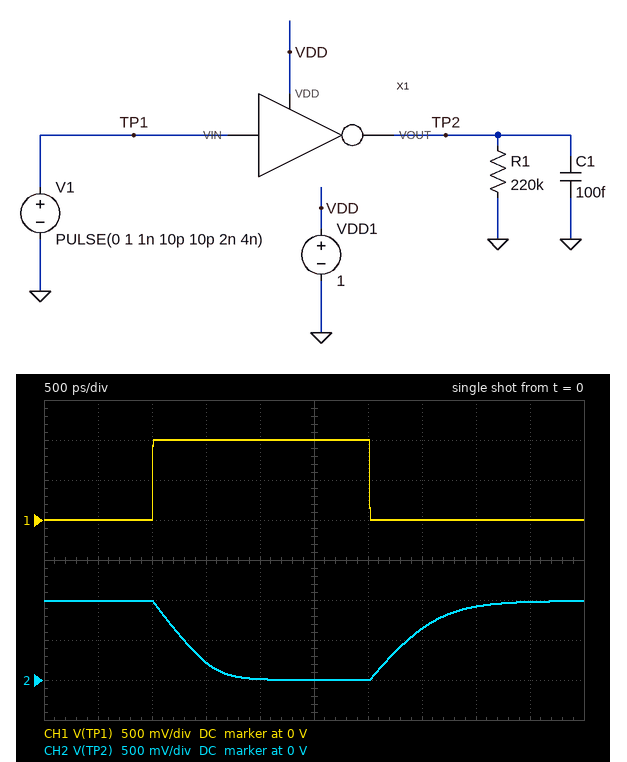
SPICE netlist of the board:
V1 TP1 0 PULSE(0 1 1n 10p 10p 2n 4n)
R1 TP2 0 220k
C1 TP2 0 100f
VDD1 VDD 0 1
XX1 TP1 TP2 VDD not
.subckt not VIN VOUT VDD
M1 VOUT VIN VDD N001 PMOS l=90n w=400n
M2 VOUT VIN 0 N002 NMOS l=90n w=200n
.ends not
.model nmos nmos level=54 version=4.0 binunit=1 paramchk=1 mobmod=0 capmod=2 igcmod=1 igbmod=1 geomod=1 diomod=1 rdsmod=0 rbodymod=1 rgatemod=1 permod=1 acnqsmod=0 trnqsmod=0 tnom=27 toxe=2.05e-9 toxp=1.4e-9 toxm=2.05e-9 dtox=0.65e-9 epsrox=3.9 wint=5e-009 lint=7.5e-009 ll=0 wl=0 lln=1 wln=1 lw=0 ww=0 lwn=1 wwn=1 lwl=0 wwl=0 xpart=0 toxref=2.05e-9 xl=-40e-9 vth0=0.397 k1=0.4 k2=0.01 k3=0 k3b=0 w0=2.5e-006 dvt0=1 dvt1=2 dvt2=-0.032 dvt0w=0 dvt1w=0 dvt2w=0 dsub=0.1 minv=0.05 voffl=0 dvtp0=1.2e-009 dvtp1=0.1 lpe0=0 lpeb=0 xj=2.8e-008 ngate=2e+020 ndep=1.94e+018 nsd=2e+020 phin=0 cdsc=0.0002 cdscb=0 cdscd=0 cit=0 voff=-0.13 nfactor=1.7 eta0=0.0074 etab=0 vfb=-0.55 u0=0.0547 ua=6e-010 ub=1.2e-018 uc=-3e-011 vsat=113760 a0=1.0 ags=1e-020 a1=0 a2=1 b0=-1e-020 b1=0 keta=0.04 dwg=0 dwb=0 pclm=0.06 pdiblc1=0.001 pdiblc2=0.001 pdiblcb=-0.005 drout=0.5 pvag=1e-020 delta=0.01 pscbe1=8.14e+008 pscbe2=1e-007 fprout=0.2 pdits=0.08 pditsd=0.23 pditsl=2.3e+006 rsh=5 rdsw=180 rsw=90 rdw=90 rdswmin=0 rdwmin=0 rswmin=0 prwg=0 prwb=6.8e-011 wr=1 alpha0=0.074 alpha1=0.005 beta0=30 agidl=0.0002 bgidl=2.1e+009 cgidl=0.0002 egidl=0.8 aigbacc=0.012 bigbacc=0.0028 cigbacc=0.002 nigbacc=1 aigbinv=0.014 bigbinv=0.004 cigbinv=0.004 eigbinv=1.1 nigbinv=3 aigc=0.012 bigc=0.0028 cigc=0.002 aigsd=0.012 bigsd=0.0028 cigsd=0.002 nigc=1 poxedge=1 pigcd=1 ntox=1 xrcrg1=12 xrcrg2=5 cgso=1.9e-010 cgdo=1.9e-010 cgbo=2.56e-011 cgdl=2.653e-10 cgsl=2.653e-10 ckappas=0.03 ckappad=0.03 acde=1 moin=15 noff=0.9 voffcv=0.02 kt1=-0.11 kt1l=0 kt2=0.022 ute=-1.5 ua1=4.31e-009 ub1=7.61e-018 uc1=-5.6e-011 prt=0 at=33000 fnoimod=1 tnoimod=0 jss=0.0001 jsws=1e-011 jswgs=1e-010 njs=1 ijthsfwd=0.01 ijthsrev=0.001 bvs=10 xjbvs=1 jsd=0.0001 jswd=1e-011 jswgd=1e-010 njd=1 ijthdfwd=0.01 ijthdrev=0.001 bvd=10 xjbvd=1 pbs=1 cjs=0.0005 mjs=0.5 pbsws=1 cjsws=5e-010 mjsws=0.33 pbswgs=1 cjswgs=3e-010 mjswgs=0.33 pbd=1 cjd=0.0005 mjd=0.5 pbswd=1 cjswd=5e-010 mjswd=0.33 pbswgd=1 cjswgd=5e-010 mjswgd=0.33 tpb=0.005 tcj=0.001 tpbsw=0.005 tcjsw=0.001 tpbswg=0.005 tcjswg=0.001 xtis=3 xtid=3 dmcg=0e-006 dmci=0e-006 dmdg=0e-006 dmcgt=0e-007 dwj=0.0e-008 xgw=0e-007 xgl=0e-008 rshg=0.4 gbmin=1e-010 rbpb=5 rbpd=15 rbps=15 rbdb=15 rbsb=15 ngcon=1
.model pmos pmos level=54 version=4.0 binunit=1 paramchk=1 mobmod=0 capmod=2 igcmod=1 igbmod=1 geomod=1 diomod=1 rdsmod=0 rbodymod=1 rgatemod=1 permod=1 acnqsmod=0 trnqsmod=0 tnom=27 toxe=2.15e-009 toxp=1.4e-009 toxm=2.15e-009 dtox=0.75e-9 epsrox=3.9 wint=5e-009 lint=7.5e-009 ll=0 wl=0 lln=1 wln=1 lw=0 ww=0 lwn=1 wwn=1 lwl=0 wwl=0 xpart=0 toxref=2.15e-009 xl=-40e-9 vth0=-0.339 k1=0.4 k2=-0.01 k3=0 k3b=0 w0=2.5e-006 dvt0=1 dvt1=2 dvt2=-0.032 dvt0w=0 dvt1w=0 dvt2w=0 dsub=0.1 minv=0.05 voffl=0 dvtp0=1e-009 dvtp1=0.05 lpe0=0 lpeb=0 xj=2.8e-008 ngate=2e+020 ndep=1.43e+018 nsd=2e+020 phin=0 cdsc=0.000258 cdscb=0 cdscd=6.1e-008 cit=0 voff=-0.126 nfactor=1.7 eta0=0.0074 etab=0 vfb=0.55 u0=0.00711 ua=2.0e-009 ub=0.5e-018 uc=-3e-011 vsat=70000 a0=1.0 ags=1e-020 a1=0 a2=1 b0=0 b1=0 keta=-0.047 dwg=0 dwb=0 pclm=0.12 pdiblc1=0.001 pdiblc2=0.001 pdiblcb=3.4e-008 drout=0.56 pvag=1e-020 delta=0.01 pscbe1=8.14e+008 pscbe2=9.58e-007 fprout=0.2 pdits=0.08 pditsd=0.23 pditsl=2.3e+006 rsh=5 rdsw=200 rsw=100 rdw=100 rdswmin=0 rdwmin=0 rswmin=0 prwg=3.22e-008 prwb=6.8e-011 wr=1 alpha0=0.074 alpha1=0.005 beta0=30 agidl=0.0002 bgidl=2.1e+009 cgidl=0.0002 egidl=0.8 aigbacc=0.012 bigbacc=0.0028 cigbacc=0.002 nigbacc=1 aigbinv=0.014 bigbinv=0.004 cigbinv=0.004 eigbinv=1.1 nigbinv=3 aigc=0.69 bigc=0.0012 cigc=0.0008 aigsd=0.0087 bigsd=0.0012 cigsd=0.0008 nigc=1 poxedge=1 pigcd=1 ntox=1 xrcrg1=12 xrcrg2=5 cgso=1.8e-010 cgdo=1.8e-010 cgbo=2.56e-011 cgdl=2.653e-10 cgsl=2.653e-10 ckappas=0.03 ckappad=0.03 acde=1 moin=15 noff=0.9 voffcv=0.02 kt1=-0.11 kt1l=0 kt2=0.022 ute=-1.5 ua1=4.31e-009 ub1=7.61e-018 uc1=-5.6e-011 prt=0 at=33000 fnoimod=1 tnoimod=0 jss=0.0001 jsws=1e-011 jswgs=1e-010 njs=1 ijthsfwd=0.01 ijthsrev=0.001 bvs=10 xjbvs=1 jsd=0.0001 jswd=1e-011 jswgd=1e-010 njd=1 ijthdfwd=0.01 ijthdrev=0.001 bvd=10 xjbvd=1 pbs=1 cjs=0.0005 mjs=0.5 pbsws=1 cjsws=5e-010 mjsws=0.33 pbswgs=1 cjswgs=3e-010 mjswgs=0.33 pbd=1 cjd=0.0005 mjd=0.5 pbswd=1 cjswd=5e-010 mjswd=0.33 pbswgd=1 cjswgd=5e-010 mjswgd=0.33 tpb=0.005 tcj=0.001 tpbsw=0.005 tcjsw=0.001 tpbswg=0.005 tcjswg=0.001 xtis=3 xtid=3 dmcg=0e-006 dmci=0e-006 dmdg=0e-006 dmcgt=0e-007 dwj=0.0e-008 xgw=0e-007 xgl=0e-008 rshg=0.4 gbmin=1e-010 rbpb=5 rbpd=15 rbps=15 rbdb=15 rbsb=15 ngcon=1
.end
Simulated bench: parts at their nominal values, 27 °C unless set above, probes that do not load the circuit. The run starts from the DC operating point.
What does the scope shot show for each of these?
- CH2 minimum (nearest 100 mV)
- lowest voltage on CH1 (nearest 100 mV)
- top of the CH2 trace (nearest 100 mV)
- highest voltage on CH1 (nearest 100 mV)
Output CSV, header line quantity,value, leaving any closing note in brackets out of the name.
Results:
quantity,value
CH2 minimum,0 V
lowest voltage on CH1,0 V
top of the CH2 trace,1.0 V
highest voltage on CH1,1.0 V
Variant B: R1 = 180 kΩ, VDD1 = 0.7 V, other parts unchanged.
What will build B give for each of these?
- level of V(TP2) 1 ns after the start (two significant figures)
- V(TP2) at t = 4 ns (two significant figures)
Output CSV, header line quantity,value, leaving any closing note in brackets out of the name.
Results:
quantity,value
level of V(TP2) 1 ns after the start,680 mV
V(TP2) at t = 4 ns,520 mV
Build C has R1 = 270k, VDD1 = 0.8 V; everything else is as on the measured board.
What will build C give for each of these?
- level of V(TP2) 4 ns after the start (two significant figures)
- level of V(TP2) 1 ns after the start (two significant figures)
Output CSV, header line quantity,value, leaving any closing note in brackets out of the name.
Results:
quantity,value
level of V(TP2) 4 ns after the start,670 mV
level of V(TP2) 1 ns after the start,790 mV
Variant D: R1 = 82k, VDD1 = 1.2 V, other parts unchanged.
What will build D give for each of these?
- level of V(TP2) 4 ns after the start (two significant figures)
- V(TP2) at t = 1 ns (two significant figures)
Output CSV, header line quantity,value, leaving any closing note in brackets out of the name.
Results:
quantity,value
level of V(TP2) 4 ns after the start,1.1 V
V(TP2) at t = 1 ns,1.2 V
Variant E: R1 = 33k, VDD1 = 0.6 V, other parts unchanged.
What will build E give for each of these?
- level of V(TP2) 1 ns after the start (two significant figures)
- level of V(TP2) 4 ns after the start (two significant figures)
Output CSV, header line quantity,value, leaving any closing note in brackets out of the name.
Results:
quantity,value
level of V(TP2) 1 ns after the start,500 mV
level of V(TP2) 4 ns after the start,330 mV
